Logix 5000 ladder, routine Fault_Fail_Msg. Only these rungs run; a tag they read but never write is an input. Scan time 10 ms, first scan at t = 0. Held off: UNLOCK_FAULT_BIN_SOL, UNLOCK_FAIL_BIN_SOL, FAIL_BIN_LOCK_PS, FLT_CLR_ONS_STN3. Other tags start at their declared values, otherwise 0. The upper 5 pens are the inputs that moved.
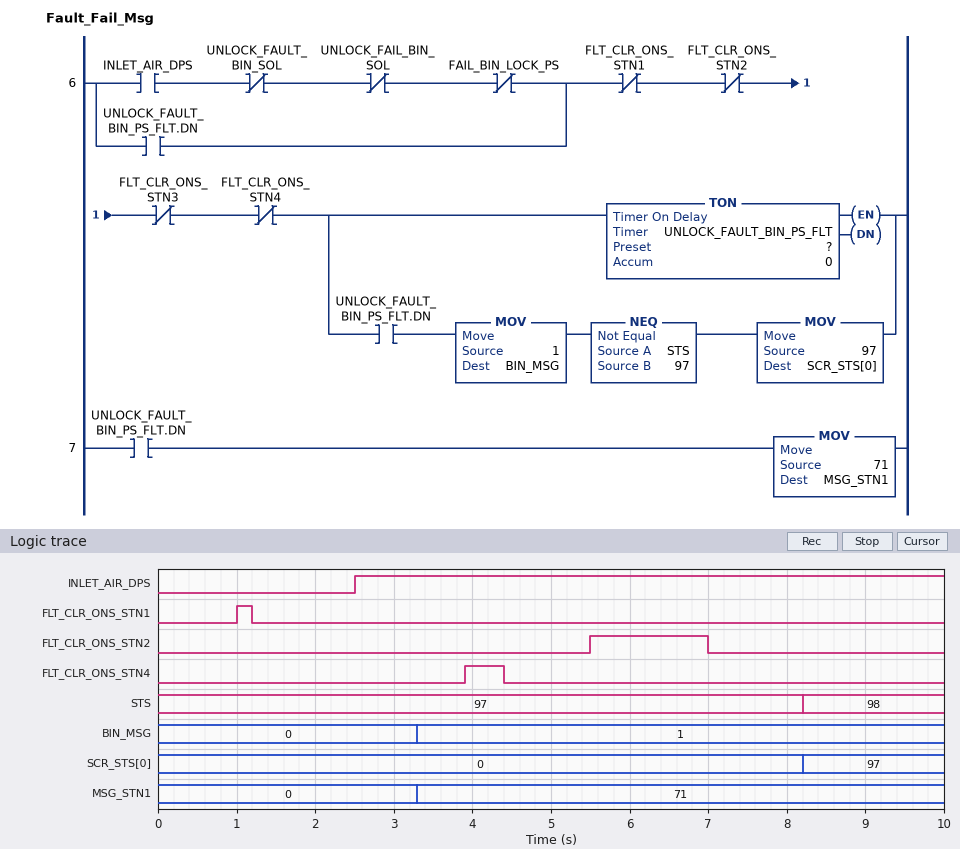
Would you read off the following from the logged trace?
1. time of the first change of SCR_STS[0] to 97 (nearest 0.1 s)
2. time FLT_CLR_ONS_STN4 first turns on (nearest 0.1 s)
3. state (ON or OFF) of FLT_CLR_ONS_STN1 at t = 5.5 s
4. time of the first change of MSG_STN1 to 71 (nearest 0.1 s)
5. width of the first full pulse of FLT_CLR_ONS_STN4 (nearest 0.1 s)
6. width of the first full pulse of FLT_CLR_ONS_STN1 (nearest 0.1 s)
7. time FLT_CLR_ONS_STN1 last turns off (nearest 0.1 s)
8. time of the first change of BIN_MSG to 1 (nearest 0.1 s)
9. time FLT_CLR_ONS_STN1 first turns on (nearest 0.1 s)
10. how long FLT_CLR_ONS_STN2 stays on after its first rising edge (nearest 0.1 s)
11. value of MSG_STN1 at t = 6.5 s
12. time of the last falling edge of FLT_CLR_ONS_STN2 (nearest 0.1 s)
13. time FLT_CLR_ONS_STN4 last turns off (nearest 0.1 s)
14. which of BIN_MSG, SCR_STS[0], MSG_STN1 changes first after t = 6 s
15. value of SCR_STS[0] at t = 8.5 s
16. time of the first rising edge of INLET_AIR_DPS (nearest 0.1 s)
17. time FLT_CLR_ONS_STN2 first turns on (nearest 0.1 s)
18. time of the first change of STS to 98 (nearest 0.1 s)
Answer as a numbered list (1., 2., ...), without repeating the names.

1. 8.2 s
2. 3.9 s
3. OFF
4. 3.3 s
5. 0.5 s
6. 0.2 s
7. 1.2 s
8. 3.3 s
9. 1.0 s
10. 1.5 s
11. 71
12. 7.0 s
13. 4.4 s
14. SCR_STS[0]
15. 97
16. 2.5 s
17. 5.5 s
18. 8.2 s
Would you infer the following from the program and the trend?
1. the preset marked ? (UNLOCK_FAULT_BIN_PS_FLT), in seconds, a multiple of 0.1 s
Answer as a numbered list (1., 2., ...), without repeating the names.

1. 0.8 s
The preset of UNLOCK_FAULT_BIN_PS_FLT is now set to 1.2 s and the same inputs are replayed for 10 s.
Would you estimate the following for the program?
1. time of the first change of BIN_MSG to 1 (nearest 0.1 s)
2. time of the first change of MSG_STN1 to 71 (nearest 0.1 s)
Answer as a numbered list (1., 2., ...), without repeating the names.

1. 3.7 s
2. 3.7 s
